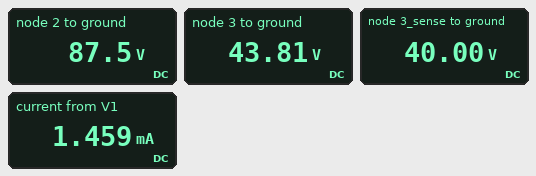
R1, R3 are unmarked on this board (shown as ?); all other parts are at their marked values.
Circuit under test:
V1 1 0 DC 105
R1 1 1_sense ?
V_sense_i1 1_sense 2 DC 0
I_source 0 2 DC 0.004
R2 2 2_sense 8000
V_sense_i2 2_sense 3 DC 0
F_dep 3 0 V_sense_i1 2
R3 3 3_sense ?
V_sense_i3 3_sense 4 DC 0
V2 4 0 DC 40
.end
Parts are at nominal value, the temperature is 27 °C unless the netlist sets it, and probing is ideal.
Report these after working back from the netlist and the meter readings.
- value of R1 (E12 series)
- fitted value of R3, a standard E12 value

12 kΩ
1.5 kΩ
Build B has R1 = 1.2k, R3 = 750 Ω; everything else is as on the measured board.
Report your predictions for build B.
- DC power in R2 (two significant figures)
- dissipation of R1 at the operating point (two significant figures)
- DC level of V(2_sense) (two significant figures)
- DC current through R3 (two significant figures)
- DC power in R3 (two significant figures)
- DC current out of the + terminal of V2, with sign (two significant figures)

460 mW
15 mW
40 V
450 µA
150 µW
-450 µA
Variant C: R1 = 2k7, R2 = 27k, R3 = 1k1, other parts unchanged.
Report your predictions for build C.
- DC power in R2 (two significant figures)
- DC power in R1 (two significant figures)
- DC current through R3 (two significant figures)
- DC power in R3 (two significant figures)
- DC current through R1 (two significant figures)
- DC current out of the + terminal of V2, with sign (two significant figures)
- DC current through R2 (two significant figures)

150 mW
7.4 mW
5.7 mA
35 mW
1.7 mA
-5.7 mA
2.3 mA
